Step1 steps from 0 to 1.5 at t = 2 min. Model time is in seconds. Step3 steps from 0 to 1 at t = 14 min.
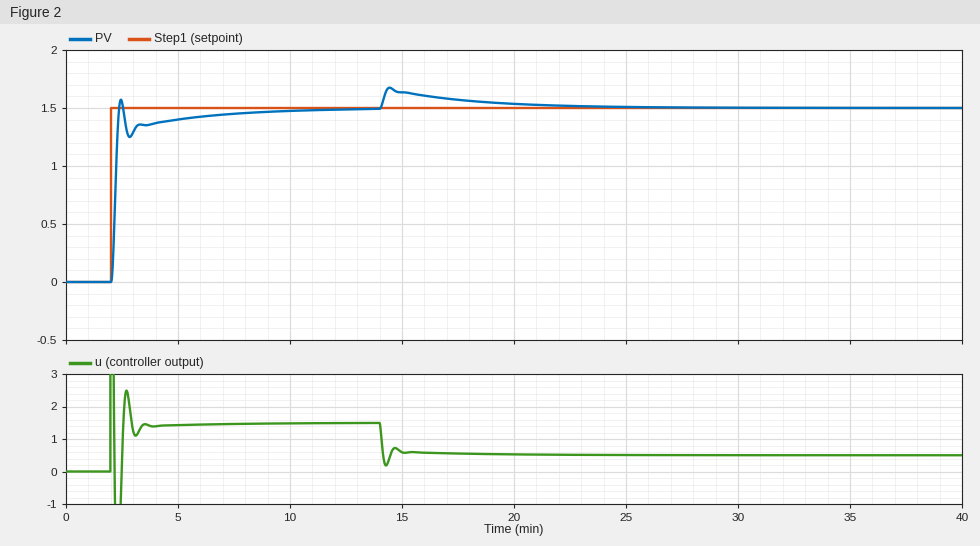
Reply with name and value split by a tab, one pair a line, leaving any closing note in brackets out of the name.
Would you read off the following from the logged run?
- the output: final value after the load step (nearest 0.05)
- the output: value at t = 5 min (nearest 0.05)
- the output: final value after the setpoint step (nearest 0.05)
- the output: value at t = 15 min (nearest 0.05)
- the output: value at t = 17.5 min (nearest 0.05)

the output: final value after the load step	1.50
the output: value at t = 5 min	1.40
the output: final value after the setpoint step	1.50
the output: value at t = 15 min	1.65
the output: value at t = 17.5 min	1.55
